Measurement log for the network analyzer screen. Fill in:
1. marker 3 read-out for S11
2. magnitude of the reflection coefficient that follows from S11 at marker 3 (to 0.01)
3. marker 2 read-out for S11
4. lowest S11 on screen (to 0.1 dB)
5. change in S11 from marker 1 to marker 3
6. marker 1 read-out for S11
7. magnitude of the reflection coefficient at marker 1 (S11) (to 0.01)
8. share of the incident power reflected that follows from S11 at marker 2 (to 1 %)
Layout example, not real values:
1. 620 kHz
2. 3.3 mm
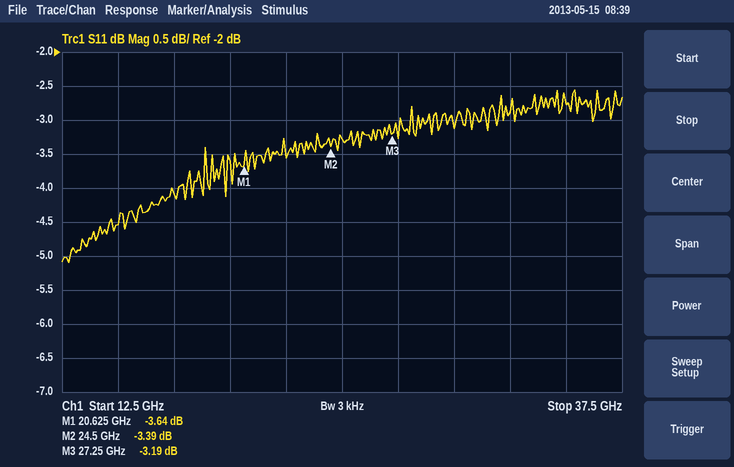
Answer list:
1. -3.19 dB
2. 0.69
3. -3.39 dB
4. -5.1 dB
5. 0.45 dB
6. -3.64 dB
7. 0.66
8. 46 %
